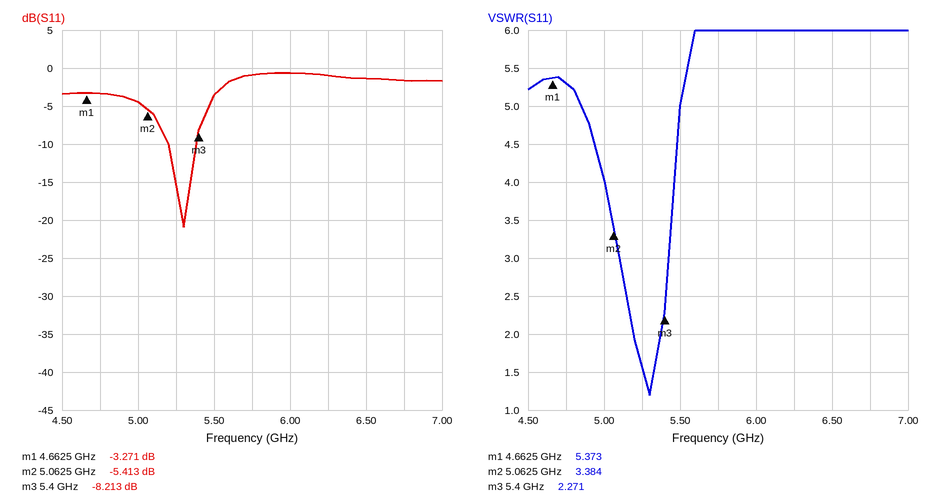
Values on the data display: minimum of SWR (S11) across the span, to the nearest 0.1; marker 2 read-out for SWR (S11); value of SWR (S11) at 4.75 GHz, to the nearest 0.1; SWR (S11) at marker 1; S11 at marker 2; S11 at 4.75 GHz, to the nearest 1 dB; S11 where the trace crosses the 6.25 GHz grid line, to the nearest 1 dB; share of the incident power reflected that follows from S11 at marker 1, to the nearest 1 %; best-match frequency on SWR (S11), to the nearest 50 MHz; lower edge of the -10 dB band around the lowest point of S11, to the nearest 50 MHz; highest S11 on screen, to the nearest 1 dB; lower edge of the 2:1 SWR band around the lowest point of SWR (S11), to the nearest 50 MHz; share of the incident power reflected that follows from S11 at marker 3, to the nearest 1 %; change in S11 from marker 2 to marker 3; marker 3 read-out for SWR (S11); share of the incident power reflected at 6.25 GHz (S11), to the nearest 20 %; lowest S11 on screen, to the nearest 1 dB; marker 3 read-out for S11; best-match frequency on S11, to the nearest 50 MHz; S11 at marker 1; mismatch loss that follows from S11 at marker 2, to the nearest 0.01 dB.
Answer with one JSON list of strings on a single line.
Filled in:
["1.2", "3.384", "5.3", "5.373", "-5.413 dB", "-3 dB", "-1 dB", "47 %", "5.30 GHz", "5.20 GHz", "-1 dB", "5.20 GHz", "15 %", "-2.800 dB", "2.271", "80 %", "-21 dB", "-8.213 dB", "5.30 GHz", "-3.271 dB", "1.47 dB"]
